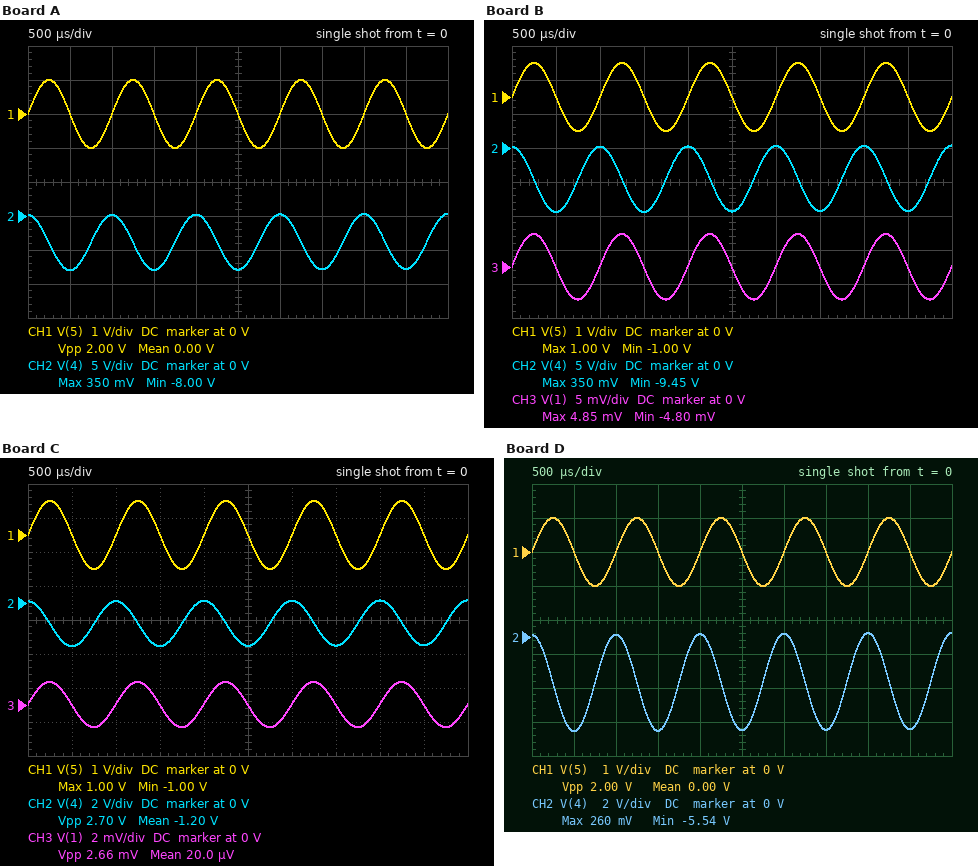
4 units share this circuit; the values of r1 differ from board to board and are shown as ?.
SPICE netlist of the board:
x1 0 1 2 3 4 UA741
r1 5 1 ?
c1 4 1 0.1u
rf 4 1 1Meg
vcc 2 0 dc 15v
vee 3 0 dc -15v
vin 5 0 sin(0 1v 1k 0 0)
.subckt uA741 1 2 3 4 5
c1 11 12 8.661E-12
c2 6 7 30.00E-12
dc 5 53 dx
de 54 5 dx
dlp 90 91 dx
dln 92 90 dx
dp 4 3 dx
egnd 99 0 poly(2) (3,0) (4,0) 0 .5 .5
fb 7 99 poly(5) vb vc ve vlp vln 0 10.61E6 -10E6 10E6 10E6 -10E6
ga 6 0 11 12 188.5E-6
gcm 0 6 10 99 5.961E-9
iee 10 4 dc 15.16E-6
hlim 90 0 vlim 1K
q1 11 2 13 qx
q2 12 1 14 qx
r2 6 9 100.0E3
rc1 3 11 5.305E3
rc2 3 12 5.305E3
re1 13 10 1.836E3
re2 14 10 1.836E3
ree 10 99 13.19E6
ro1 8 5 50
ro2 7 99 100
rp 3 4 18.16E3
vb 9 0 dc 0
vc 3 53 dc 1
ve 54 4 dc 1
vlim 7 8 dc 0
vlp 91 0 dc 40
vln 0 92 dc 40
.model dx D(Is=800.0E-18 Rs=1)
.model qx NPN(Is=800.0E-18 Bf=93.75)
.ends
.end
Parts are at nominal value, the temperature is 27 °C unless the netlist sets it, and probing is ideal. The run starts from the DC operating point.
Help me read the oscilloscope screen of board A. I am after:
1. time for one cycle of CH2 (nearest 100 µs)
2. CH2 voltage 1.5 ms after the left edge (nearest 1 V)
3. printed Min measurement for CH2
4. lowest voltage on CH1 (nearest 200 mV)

1.0 ms
-8 V
-8.00 V
-1.0 V
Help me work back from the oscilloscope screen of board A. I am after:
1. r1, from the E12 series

390 Ω
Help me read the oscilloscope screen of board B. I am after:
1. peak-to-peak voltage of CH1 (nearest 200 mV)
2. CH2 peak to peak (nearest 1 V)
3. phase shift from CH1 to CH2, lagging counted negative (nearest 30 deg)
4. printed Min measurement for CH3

2.0 V
10 V
90 deg
-4.80 mV
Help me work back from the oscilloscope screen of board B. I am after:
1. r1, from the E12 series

330 Ω
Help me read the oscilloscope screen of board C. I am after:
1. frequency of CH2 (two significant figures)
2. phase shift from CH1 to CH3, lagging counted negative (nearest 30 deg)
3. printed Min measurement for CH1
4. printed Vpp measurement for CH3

1.0 kHz
0 deg
-1.00 V
2.66 mV
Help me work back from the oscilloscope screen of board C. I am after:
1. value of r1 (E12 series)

1.2 kΩ
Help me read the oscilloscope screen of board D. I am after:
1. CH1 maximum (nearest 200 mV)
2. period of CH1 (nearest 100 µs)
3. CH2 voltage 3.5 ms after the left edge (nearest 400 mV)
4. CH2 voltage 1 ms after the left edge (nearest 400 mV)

1.0 V
1.0 ms
-5.6 V
0 V
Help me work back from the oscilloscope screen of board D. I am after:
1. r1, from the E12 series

560 Ω
